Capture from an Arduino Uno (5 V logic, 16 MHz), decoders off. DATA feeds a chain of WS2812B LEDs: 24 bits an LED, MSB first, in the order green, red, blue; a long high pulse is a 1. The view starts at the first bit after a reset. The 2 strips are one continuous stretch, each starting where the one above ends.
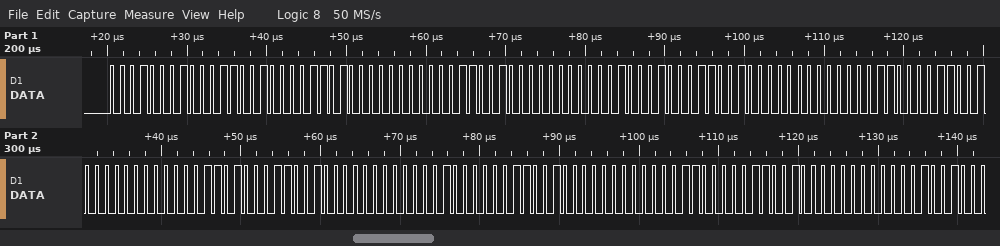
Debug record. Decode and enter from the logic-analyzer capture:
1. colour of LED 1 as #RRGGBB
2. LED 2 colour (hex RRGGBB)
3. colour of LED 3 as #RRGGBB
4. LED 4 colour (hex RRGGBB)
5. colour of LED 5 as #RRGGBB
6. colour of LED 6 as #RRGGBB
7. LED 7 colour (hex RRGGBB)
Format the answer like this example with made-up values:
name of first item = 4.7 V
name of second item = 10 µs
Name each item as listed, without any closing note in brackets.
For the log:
colour of LED 1 as #RRGGBB = #19110D
LED 2 colour = #190000
colour of LED 3 as #RRGGBB = #191100
LED 4 colour = #190600
colour of LED 5 as #RRGGBB = #190D00
colour of LED 6 as #RRGGBB = #190800
LED 7 colour = #190C00
